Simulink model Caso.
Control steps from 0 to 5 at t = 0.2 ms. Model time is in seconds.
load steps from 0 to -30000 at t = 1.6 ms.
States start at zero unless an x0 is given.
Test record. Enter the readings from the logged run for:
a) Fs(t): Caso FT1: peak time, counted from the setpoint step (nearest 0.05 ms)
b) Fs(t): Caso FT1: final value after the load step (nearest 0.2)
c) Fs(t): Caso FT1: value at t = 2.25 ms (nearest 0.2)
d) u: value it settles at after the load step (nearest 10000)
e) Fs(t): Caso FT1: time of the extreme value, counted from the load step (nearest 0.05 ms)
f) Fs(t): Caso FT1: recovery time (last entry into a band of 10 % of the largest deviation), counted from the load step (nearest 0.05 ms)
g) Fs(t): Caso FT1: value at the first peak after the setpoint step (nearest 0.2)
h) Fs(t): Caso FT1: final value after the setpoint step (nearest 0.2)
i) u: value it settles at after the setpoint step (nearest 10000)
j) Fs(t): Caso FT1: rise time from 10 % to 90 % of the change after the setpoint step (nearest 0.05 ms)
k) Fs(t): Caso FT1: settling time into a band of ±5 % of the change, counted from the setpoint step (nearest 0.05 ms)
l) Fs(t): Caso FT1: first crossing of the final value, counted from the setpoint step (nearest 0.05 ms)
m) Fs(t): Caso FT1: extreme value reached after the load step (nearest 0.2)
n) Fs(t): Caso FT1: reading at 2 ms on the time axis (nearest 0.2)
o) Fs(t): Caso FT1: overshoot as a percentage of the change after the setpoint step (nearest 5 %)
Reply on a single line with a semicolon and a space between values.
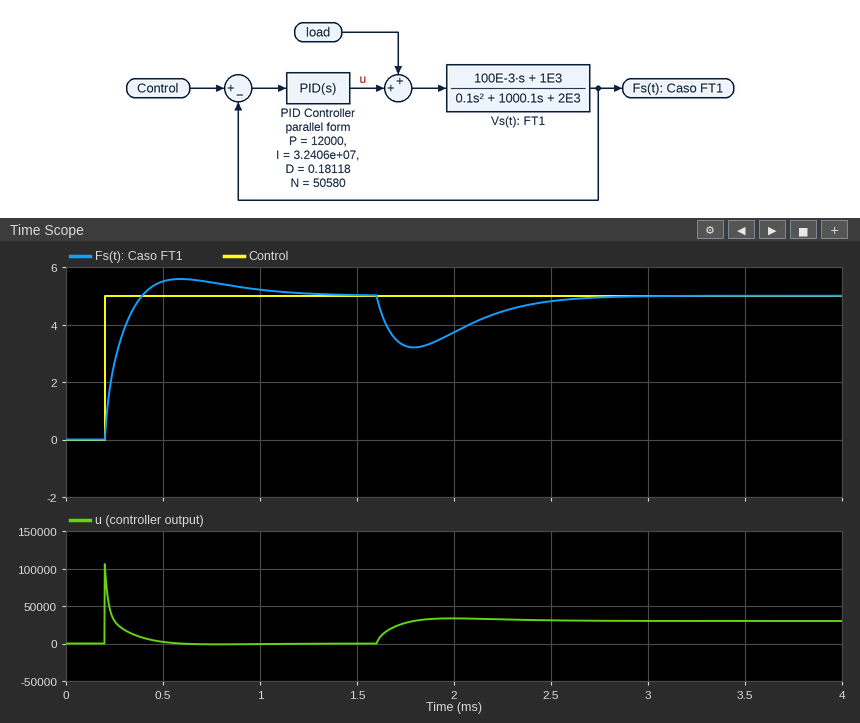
0.40 ms; 5.0; 4.4; 30000; 0.20 ms; 0.90 ms; 5.6; 5.0; 0; 0.15 ms; 0.75 ms; 0.20 ms; 3.2; 3.8; 10 %
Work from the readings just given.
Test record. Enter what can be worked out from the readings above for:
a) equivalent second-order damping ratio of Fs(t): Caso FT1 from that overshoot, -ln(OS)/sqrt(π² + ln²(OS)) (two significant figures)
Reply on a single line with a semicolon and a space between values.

0.59
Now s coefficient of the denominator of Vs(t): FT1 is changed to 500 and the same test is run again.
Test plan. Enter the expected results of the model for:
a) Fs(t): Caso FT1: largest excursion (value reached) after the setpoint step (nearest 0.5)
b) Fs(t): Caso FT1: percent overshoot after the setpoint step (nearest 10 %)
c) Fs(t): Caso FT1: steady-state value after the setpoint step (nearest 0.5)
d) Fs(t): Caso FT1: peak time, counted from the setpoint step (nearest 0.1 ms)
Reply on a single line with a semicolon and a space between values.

6.0; 20 %; 5.0; 0.3 ms
